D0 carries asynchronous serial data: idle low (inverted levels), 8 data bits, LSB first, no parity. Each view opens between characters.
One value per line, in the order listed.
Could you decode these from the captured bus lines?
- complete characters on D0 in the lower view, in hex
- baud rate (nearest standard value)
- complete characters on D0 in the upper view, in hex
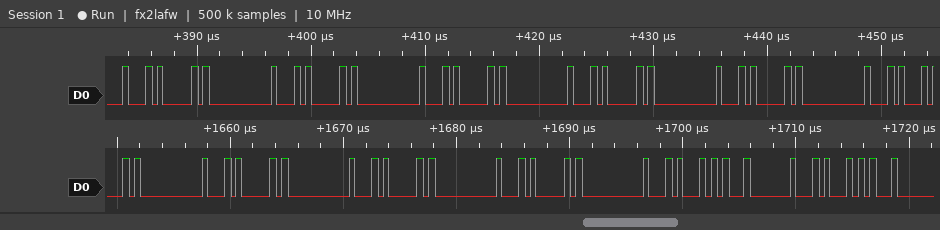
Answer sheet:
FD, D7, FD, D7, FD, D7, FD, D7, 75, D7, 75
2000000 baud
D7, FD, D7, FD, D7, FD, D7, FD, D7, FD, D7
